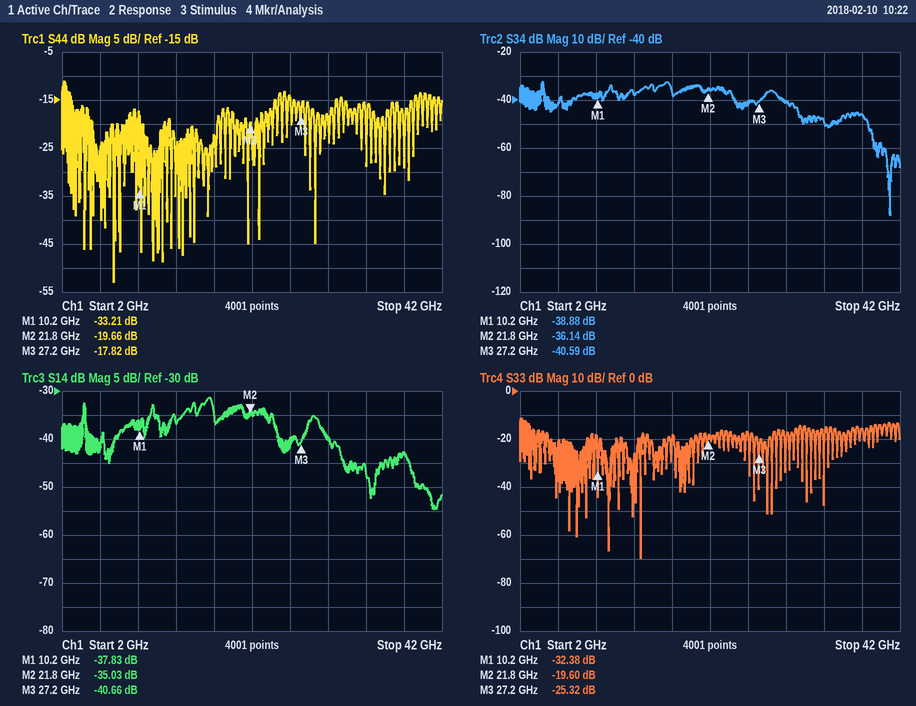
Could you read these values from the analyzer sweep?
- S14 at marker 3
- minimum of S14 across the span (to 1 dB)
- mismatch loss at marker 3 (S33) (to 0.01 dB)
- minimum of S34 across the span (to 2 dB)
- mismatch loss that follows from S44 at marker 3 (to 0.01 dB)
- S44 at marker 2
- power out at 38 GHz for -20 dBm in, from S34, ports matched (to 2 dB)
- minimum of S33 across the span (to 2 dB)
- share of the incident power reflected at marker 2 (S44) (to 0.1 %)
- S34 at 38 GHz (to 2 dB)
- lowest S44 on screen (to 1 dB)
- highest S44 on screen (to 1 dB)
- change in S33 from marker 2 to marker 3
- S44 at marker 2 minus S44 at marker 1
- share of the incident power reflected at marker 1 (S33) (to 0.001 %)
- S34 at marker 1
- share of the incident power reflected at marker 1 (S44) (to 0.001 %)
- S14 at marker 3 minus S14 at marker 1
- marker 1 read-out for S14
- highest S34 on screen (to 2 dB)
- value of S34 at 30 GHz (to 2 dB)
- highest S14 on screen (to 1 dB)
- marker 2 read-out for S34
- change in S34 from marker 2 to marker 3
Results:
-40.66 dB
-55 dB
0.01 dB
-88 dB
0.07 dB
-19.66 dB
-66 dBm
-70 dB
1.1 %
-46 dB
-53 dB
-11 dB
-5.72 dB
13.55 dB
0.058 %
-38.88 dB
0.048 %
-2.83 dB
-37.83 dB
-32 dB
-40 dB
-31 dB
-36.14 dB
-4.45 dB
